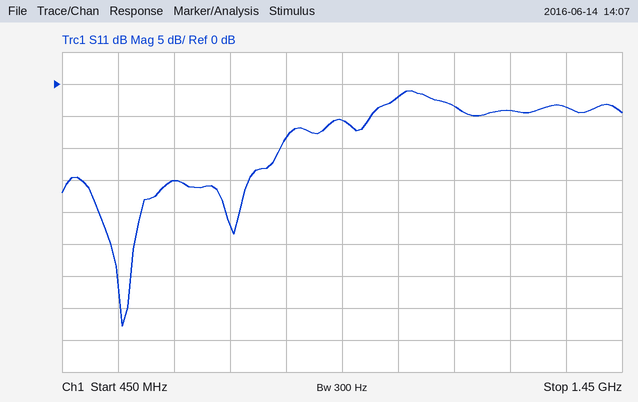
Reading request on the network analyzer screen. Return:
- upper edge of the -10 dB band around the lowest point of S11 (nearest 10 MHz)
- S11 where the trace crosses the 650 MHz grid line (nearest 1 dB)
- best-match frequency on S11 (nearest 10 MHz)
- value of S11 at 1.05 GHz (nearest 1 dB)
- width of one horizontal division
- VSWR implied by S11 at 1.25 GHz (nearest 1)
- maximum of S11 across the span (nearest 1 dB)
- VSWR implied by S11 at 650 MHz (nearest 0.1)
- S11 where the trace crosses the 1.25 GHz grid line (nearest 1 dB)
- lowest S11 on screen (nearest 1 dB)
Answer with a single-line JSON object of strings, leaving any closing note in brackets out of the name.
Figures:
{"upper edge of the -10 dB band around the lowest point of S11": "840 MHz", "S11 where the trace crosses the 650 MHz grid line": "-15 dB", "best-match frequency on S11": "560 MHz", "value of S11 at 1.05 GHz": "-2 dB", "width of one horizontal division": "100 MHz", "VSWR implied by S11 at 1.25 GHz": "4", "maximum of S11 across the span": "-1 dB", "VSWR implied by S11 at 650 MHz": "1.4", "S11 where the trace crosses the 1.25 GHz grid line": "-4 dB", "lowest S11 on screen": "-38 dB"}
